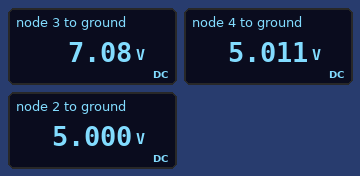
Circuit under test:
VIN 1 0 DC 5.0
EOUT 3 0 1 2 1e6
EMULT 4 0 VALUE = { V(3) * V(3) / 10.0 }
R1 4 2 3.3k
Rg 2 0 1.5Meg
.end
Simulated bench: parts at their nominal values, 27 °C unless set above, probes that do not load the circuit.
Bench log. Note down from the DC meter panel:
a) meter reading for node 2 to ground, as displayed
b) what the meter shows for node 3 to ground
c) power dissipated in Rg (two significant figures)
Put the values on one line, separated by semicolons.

5.000 V; 7.08 V; 17 µW
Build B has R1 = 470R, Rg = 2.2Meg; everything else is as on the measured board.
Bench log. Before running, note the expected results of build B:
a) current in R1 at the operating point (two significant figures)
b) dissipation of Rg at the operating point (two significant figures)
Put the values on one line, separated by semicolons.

2.3 µA; 11 µW
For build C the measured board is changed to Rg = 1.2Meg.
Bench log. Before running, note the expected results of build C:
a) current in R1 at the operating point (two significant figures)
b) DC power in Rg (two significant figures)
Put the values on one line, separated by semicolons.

4.2 µA; 21 µW
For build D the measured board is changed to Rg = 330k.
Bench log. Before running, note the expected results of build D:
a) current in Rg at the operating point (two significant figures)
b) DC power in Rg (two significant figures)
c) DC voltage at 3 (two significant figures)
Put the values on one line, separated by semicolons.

15 µA; 76 µW; 7.1 V
